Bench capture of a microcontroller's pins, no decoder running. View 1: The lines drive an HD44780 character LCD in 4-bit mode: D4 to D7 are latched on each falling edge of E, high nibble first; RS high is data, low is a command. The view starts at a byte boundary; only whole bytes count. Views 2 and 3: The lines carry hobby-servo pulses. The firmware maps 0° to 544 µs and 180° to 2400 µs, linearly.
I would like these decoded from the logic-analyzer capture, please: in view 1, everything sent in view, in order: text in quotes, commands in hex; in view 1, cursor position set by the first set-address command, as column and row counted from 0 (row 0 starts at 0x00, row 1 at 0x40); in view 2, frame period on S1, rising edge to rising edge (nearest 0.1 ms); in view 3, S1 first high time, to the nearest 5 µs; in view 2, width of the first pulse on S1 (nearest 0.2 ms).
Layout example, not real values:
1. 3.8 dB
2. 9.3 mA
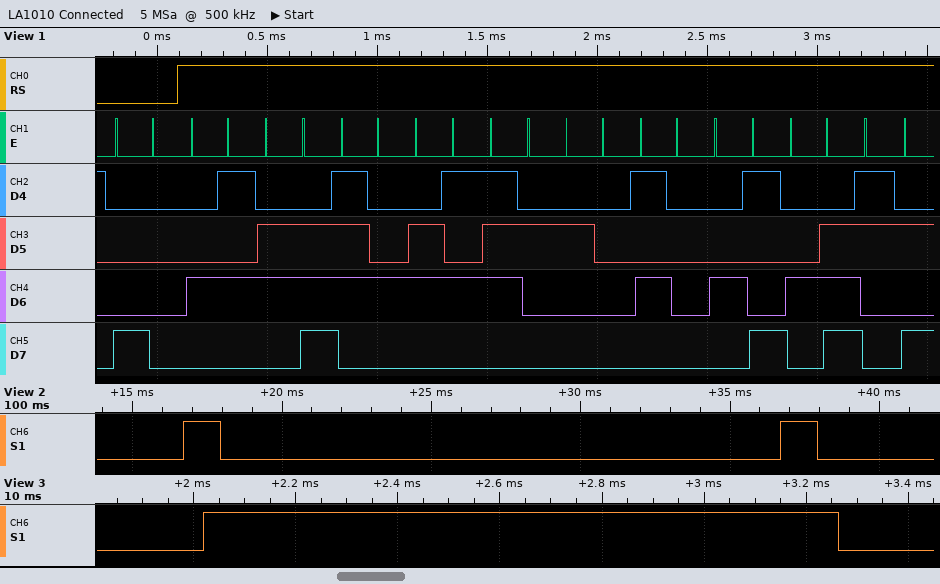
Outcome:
1. 0x80 "Enter PIN:"
2. column 0, row 0
3. 20.0 ms
4. 1245 µs
5. 1.2 ms
